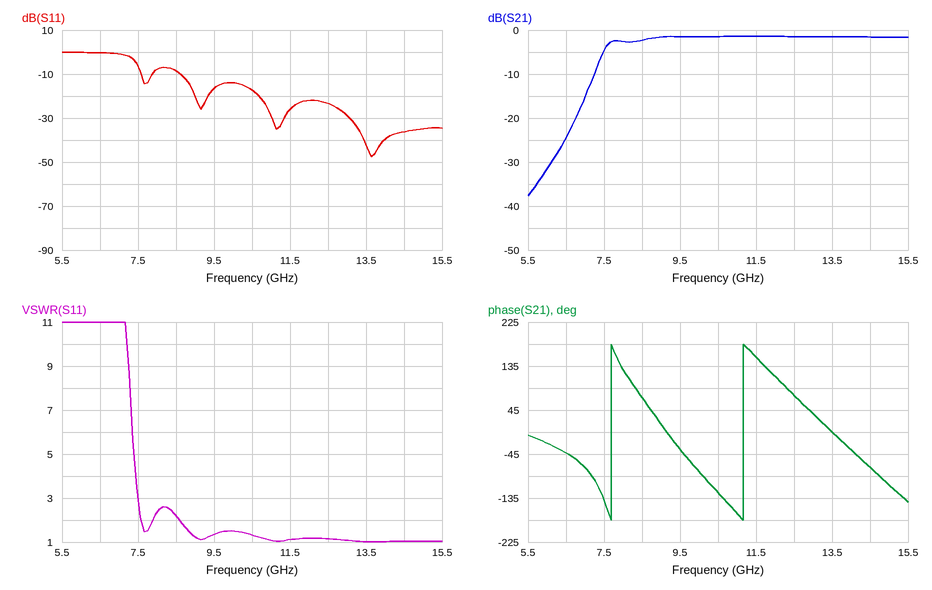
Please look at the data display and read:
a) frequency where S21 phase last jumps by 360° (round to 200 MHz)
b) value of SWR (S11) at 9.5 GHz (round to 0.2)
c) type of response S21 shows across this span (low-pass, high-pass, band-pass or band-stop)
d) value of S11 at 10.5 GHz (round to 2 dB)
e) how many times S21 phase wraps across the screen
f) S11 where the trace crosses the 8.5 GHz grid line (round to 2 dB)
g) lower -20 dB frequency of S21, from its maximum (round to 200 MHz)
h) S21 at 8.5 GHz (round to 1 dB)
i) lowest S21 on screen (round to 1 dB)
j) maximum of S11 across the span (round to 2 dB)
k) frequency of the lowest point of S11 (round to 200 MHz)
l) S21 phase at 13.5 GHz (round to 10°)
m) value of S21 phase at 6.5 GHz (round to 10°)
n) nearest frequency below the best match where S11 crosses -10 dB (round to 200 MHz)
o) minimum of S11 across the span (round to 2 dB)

11.2 GHz
1.4
high-pass
-18 dB
2
-8 dB
6.6 GHz
-2 dB
-38 dB
0 dB
13.6 GHz
0°
-40°
8.6 GHz
-48 dB
